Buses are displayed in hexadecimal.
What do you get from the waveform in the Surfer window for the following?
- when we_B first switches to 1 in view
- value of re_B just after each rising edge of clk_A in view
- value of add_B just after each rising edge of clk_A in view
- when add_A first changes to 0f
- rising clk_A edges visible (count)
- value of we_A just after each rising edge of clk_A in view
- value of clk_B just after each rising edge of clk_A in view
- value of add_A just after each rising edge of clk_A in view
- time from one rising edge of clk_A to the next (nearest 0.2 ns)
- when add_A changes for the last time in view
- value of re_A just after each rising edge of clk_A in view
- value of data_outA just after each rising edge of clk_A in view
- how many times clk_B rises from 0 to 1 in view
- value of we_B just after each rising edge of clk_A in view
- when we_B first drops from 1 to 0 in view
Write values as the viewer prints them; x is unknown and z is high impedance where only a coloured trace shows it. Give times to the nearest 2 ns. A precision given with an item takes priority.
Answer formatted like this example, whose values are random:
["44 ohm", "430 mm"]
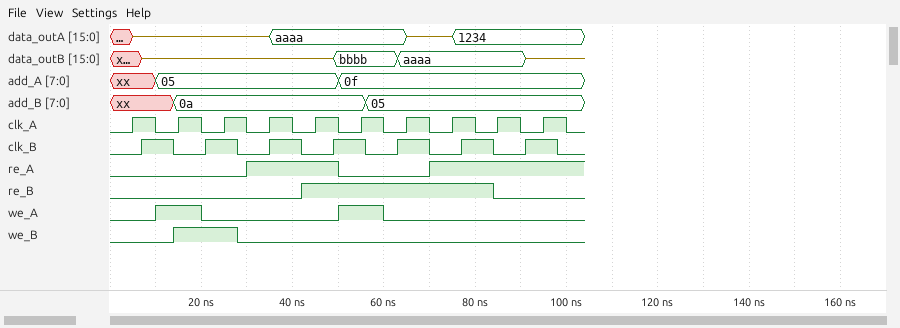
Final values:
["14 ns", "0 0 0 0 1 1 1 1 0 0", "xx, 0a, 0a, 0a, 0a, 0a, 05, 05, 05, 05", "50 ns", "10", "0 1 0 0 0 1 0 0 0 0", "0 0 1 1 0 1 1 0 0 1", "xx, 05, 05, 05, 05, 0f, 0f, 0f, 0f, 0f", "10 ns", "50 ns", "0 0 0 1 1 0 0 1 1 1", "z, z, z, aaaa, aaaa, aaaa, z, 1234, 1234, 1234", "7", "0 1 1 0 0 0 0 0 0 0", "28 ns"]
